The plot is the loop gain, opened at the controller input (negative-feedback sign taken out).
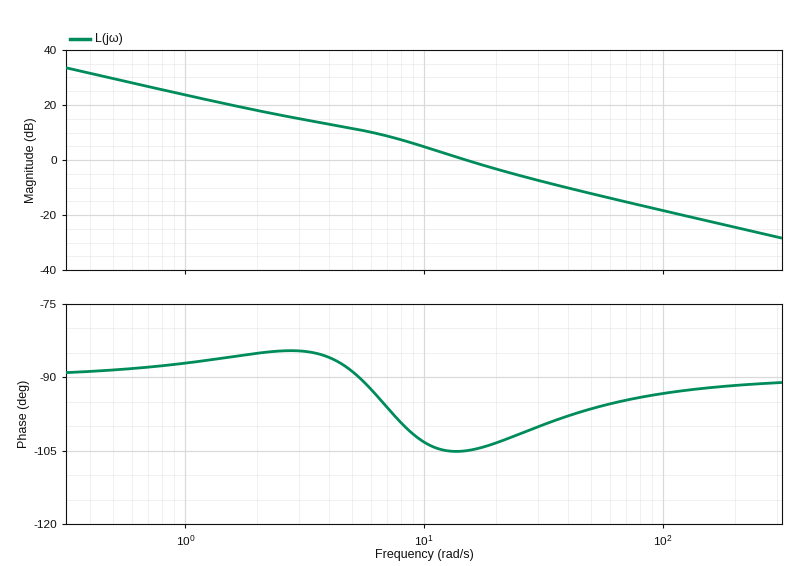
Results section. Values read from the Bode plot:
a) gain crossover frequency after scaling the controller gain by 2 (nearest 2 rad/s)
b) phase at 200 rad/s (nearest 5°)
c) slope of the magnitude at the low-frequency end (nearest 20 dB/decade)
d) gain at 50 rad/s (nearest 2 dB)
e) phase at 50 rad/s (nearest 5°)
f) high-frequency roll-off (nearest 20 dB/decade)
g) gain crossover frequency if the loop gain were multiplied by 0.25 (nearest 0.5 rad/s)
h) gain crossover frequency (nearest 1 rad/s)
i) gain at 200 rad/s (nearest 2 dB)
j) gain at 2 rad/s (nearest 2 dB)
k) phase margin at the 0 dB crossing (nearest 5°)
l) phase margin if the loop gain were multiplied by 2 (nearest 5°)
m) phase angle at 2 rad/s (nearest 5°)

26 rad/s
-90°
-20 dB/decade
-12 dB
-95°
-20 dB/decade
4.5 rad/s
15 rad/s
-24 dB
18 dB
75°
80°
-85°
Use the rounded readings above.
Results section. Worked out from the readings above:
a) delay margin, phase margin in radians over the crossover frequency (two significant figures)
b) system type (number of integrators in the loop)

0.087 s
1
